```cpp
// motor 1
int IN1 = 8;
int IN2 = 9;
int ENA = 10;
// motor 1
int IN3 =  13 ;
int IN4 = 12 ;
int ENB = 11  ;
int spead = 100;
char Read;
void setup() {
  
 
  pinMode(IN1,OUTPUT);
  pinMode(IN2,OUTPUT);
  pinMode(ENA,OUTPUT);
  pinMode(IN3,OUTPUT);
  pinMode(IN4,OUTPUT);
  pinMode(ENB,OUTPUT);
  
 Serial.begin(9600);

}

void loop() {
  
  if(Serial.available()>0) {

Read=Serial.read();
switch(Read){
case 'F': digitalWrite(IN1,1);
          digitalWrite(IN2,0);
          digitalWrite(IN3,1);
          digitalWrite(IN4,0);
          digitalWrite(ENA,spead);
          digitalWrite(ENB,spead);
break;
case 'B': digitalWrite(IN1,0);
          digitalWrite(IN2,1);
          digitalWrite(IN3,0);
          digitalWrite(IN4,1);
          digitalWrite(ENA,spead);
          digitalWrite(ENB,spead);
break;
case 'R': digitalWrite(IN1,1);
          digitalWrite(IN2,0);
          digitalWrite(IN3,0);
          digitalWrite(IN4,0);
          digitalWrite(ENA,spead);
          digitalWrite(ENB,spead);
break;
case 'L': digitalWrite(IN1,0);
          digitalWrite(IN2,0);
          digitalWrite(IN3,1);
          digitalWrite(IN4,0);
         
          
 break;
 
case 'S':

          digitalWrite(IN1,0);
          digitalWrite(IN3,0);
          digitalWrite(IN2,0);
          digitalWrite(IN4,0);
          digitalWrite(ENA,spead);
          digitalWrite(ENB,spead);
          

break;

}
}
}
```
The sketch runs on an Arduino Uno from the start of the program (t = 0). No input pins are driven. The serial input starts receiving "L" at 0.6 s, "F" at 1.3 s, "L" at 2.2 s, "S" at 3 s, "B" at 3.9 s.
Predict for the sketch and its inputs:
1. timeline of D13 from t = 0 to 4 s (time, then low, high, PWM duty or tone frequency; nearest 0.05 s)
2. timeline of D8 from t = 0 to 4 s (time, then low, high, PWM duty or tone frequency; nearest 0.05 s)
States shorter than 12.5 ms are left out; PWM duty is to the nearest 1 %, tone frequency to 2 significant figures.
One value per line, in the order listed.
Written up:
0 s low; 0.6 s high; 3 s low
0 s low; 1.3 s high; 2.2 s low
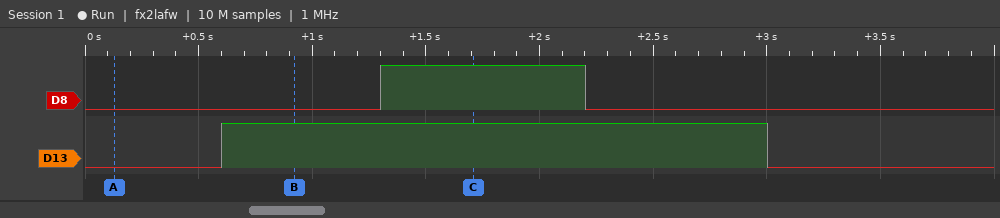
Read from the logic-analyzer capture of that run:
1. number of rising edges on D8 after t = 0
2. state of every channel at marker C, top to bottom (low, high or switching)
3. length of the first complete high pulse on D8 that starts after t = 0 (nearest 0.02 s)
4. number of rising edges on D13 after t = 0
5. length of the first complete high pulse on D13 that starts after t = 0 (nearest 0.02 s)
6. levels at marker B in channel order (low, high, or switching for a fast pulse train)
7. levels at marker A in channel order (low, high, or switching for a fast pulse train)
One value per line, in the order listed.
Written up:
1
D8 high, D13 high
0.90 s
1
2.40 s
D8 low, D13 high
D8 low, D13 low
